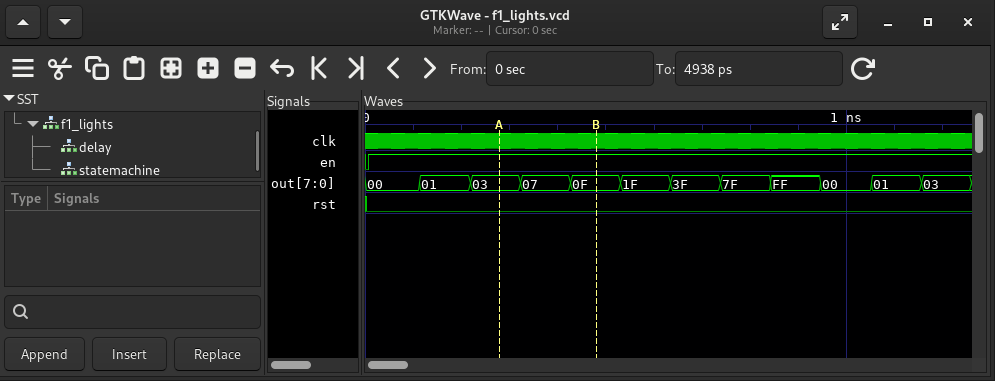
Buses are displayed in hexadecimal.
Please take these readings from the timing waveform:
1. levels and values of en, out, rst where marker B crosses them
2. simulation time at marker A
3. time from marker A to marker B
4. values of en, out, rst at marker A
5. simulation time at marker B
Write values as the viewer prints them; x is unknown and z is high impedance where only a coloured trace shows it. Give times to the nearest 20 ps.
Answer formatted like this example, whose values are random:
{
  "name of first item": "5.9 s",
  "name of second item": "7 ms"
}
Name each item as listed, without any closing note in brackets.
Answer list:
{
  "levels and values of en, out, rst where marker B crosses them": "en=1, out=0F, rst=0",
  "simulation time at marker A": "280 ps",
  "time from marker A to marker B": "200 ps",
  "values of en, out, rst at marker A": "en=1, out=03, rst=0",
  "simulation time at marker B": "480 ps"
}
